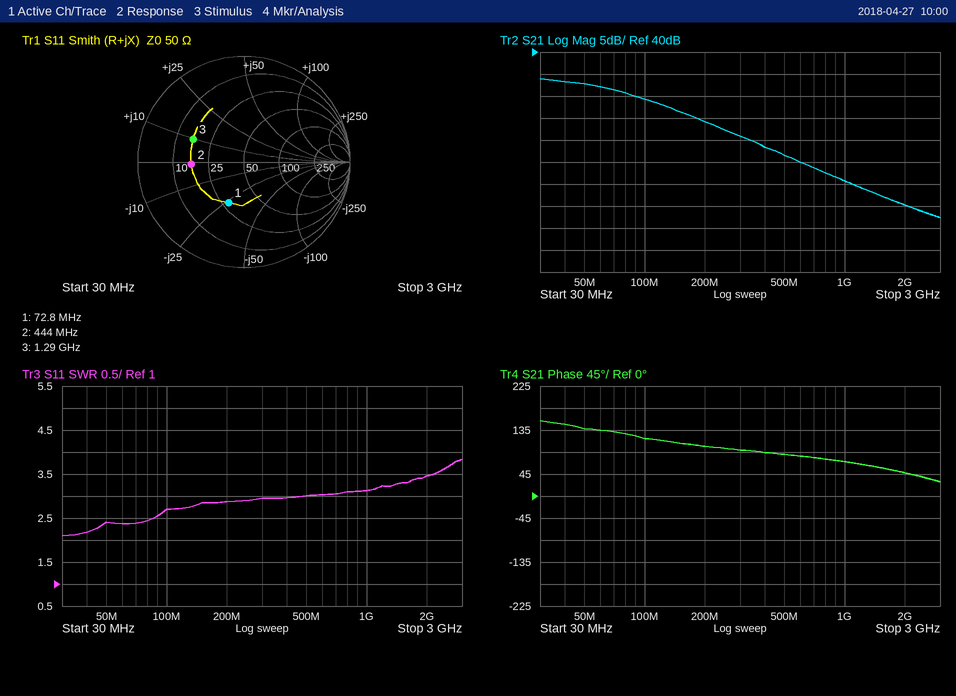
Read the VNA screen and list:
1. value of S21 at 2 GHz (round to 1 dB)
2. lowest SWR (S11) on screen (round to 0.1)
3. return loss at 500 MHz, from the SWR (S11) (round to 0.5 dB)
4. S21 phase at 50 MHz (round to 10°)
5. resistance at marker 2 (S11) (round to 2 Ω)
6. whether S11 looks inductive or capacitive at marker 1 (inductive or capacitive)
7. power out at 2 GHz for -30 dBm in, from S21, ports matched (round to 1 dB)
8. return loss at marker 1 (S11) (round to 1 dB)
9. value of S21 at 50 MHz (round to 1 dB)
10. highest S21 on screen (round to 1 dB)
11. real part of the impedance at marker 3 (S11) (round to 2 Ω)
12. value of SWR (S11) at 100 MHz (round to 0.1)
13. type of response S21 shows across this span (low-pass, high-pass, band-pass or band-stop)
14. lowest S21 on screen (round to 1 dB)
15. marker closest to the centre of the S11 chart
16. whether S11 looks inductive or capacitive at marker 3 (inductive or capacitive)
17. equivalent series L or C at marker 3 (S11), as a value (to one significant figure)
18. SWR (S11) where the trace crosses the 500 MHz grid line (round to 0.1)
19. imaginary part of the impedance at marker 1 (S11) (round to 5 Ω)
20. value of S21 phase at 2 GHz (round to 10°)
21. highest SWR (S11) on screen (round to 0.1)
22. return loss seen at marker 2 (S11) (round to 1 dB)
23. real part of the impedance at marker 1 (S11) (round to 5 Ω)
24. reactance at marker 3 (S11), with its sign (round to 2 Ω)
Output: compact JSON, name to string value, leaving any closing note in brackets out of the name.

{"value of S21 at 2 GHz": "5 dB", "lowest SWR (S11) on screen": "2.1", "return loss at 500 MHz, from the SWR (S11)": "6.0 dB", "S21 phase at 50 MHz": "140°", "resistance at marker 2 (S11)": "16 Ω", "whether S11 looks inductive or capacitive at marker 1": "capacitive", "power out at 2 GHz for -30 dBm in, from S21, ports matched": "-25 dBm", "return loss at marker 1 (S11)": "8 dB", "value of S21 at 50 MHz": "33 dB", "highest S21 on screen": "34 dB", "real part of the impedance at marker 3 (S11)": "16 Ω", "value of SWR (S11) at 100 MHz": "2.7", "type of response S21 shows across this span": "low-pass", "lowest S21 on screen": "2 dB", "marker closest to the centre of the S11 chart": "marker 1", "whether S11 looks inductive or capacitive at marker 3": "inductive", "equivalent series L or C at marker 3 (S11), as a value": "1 nH", "SWR (S11) where the trace crosses the 500 MHz grid line": "3.0", "imaginary part of the impedance at marker 1 (S11)": "-25 Ω", "value of S21 phase at 2 GHz": "50°", "highest SWR (S11) on screen": "3.8", "return loss seen at marker 2 (S11)": "6 dB", "real part of the impedance at marker 1 (S11)": "30 Ω", "reactance at marker 3 (S11), with its sign": "+10 Ω"}
